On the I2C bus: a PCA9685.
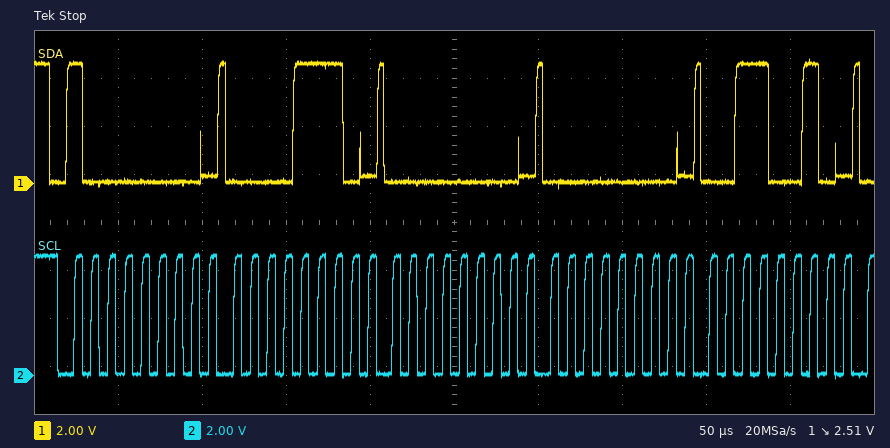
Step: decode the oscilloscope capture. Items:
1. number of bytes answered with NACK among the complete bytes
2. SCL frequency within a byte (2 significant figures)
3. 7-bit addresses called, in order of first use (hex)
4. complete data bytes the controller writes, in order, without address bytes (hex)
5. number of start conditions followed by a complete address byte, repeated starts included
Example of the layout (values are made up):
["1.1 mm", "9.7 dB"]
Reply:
["0", "100 kHz", "0x40", "0E 00 00 32", "1"]
